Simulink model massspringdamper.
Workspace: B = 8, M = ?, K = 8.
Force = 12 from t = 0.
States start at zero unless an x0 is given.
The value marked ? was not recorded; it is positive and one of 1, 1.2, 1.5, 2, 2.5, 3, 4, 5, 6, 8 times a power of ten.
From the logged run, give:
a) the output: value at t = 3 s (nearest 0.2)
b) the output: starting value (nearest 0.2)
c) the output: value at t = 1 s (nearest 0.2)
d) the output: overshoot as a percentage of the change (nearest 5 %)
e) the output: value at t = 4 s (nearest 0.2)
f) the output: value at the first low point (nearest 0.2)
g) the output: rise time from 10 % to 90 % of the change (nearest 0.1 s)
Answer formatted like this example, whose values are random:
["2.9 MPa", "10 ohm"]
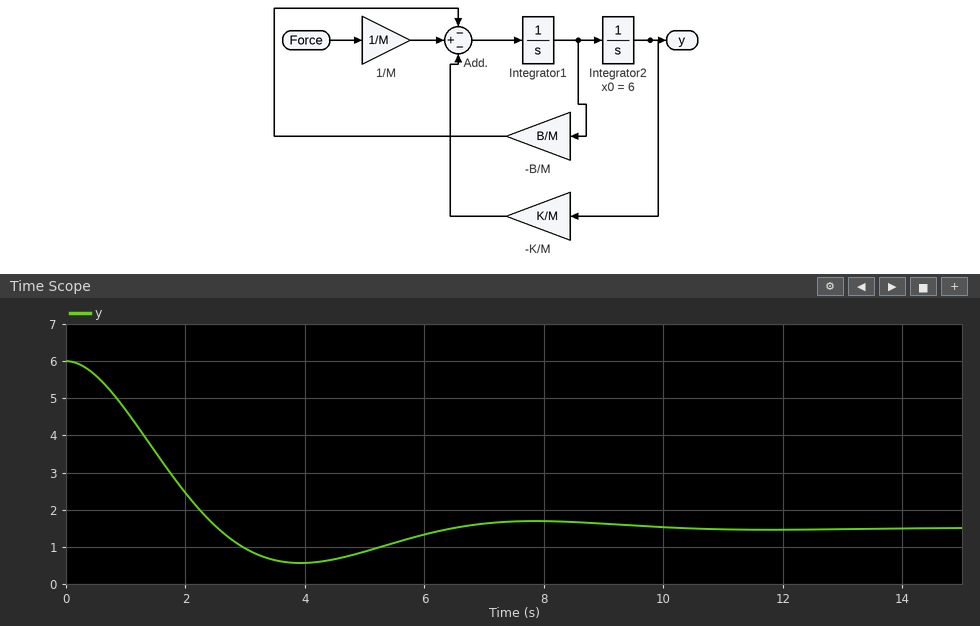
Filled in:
["1.0", "6.0", "4.6", "20 %", "0.6", "0.6", "1.7 s"]
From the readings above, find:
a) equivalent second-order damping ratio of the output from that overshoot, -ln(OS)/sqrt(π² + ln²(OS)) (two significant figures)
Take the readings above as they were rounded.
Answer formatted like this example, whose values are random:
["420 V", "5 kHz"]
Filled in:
["0.46"]
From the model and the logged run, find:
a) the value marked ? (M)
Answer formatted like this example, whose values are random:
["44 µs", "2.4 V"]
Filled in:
["10"]
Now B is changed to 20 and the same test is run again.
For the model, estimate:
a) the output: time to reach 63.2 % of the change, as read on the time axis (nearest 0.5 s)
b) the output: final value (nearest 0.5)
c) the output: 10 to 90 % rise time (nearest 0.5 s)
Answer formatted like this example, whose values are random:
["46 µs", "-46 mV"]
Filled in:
["2.5 s", "1.5", "4.5 s"]
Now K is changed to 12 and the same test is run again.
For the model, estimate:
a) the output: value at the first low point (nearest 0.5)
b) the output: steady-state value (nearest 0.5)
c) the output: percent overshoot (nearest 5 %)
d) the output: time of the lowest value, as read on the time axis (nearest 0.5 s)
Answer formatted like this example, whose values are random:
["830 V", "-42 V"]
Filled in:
["-0.5", "1.0", "30 %", "3.0 s"]
